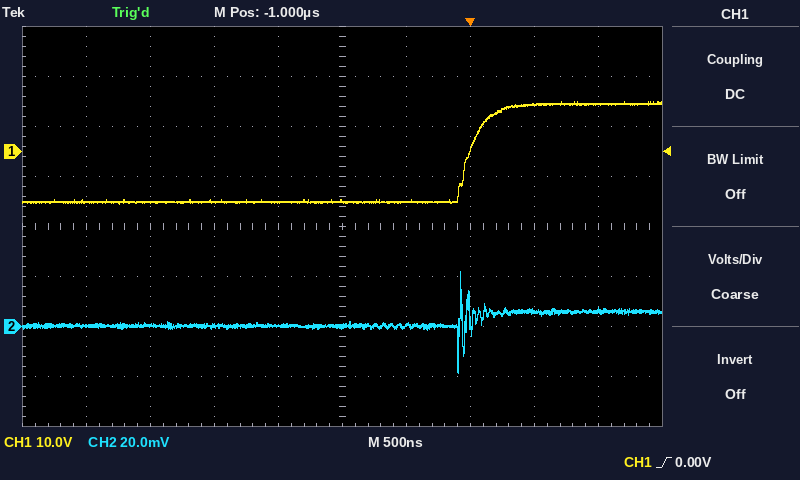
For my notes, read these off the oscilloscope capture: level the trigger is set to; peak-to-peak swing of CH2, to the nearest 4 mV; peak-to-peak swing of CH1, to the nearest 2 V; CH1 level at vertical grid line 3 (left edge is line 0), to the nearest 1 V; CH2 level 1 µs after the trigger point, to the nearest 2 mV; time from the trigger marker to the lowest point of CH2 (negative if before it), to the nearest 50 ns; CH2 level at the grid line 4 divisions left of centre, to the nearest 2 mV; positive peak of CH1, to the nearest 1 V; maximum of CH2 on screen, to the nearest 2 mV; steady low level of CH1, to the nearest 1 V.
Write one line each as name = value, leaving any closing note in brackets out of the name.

level the trigger is set to = 0.00 V
peak-to-peak swing of CH2, to the nearest 4 mV = 40 mV
peak-to-peak swing of CH1, to the nearest 2 V = 20 V
CH1 level at vertical grid line 3 (left edge is line 0), to the nearest 1 V = -10 V
CH2 level 1 µs after the trigger point, to the nearest 2 mV = 6 mV
time from the trigger marker to the lowest point of CH2 (negative if before it), to the nearest 50 ns = -100 ns
CH2 level at the grid line 4 divisions left of centre, to the nearest 2 mV = 0 mV
positive peak of CH1, to the nearest 1 V = 10 V
maximum of CH2 on screen, to the nearest 2 mV = 22 mV
steady low level of CH1, to the nearest 1 V = -10 V
